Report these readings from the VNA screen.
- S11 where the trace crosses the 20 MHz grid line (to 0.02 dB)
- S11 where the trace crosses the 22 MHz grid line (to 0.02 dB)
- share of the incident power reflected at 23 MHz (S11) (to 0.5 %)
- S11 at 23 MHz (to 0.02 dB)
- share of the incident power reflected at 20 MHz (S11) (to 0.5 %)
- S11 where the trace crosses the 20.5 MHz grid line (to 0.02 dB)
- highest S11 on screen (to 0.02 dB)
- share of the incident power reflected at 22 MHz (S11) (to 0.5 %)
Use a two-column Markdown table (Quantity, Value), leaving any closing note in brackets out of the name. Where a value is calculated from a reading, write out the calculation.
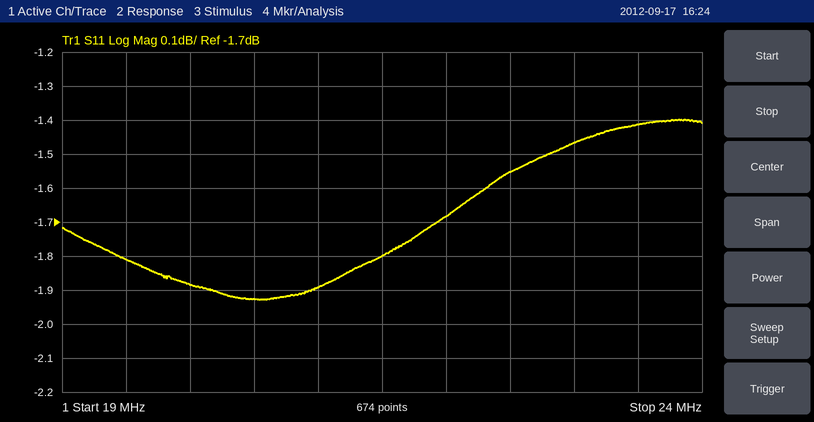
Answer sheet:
| Quantity | Value |
|---|---|
| S11 where the trace crosses the 20 MHz grid line | -1.88 dB |
| S11 where the trace crosses the 22 MHz grid line | -1.68 dB |
| share of the incident power reflected at 23 MHz (S11) | 10^(-1.46/10) ≈ 71.4 %, so 71.5 % to the nearest 0.5 % |
| S11 at 23 MHz | -1.46 dB |
| share of the incident power reflected at 20 MHz (S11) | 10^(-1.88/10) ≈ 64.9 %, so 65.0 % to the nearest 0.5 % |
| S11 where the trace crosses the 20.5 MHz grid line | -1.92 dB |
| highest S11 on screen | -1.40 dB |
| share of the incident power reflected at 22 MHz (S11) | 10^(-1.68/10) ≈ 67.9 %, so 68.0 % to the nearest 0.5 % |
